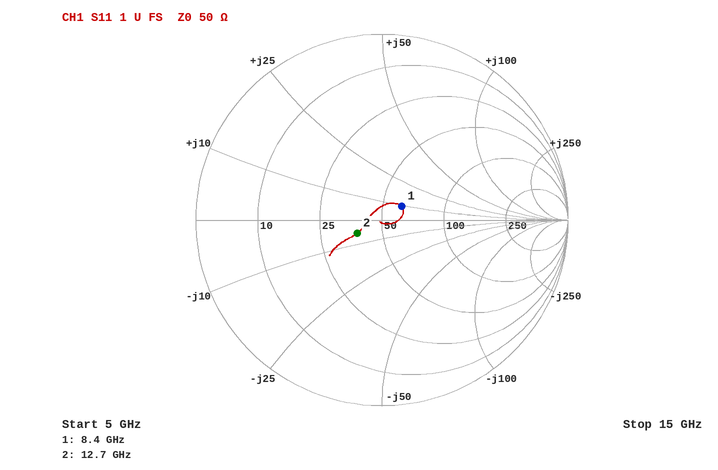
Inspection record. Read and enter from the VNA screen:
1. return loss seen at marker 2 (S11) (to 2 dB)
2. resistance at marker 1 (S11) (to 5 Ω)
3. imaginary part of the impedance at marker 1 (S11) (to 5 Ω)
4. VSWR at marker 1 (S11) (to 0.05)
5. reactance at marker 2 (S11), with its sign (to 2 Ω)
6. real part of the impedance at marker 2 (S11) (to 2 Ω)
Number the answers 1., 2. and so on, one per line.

1. 16 dB
2. 60 Ω
3. +10 Ω
4. 1.30
5. -6 Ω
6. 38 Ω
